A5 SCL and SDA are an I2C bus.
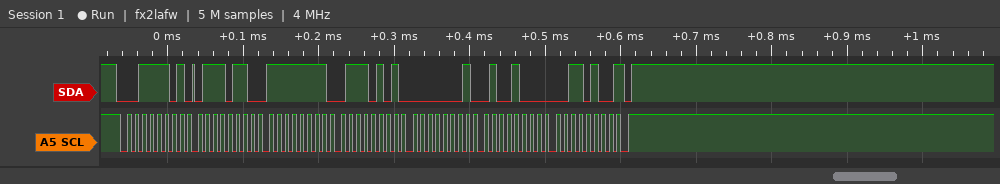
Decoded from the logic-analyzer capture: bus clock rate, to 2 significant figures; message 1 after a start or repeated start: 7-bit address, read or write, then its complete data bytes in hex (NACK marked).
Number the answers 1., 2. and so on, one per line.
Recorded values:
1. 100 kHz
2. 0x1E read: 76 FF 75 01 48 34 NACK
